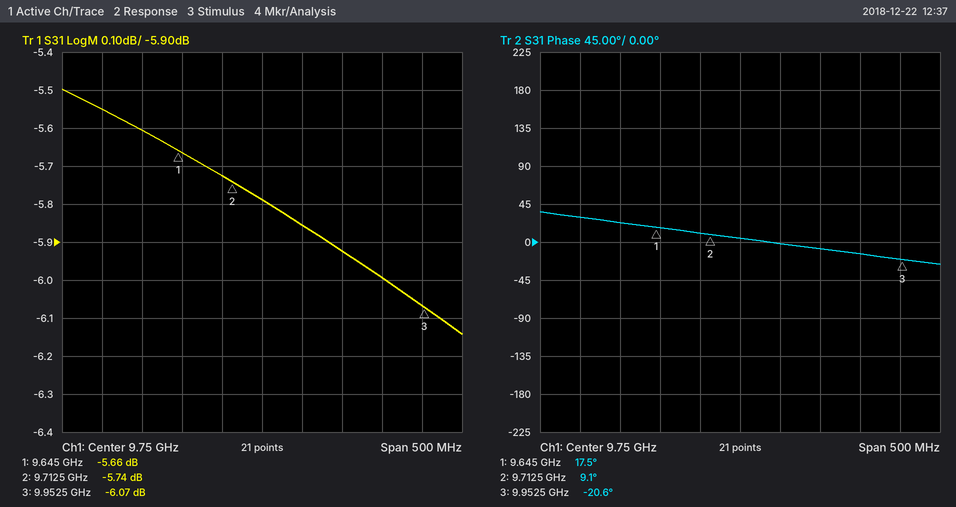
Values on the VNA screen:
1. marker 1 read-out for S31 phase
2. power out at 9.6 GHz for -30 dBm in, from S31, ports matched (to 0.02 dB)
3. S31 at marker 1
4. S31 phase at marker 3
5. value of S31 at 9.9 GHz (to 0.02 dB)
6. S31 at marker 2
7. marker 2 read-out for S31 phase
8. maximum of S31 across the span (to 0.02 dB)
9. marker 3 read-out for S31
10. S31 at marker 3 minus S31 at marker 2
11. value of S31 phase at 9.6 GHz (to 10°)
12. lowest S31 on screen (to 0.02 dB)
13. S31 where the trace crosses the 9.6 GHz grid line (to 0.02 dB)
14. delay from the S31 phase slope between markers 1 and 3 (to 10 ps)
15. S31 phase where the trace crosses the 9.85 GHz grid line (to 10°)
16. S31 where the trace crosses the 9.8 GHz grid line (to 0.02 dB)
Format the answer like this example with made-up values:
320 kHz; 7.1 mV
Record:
17.5°; -35.60 dBm; -5.66 dB; -20.6°; -6.00 dB; -5.74 dB; 9.1°; -5.50 dB; -6.07 dB; -0.33 dB; 20°; -6.14 dB; -5.60 dB; 340 ps; -10°; -5.86 dB
